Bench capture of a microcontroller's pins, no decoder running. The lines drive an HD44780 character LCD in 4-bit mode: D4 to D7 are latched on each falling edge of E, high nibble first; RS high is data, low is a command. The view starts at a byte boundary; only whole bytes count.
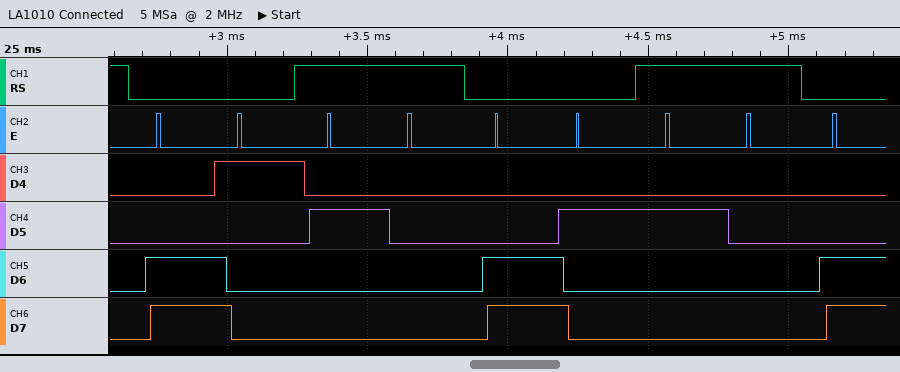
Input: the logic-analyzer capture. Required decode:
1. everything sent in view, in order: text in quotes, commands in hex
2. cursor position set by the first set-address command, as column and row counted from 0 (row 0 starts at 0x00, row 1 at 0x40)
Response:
0xC1 " " 0xC2 " "
column 1, row 1
